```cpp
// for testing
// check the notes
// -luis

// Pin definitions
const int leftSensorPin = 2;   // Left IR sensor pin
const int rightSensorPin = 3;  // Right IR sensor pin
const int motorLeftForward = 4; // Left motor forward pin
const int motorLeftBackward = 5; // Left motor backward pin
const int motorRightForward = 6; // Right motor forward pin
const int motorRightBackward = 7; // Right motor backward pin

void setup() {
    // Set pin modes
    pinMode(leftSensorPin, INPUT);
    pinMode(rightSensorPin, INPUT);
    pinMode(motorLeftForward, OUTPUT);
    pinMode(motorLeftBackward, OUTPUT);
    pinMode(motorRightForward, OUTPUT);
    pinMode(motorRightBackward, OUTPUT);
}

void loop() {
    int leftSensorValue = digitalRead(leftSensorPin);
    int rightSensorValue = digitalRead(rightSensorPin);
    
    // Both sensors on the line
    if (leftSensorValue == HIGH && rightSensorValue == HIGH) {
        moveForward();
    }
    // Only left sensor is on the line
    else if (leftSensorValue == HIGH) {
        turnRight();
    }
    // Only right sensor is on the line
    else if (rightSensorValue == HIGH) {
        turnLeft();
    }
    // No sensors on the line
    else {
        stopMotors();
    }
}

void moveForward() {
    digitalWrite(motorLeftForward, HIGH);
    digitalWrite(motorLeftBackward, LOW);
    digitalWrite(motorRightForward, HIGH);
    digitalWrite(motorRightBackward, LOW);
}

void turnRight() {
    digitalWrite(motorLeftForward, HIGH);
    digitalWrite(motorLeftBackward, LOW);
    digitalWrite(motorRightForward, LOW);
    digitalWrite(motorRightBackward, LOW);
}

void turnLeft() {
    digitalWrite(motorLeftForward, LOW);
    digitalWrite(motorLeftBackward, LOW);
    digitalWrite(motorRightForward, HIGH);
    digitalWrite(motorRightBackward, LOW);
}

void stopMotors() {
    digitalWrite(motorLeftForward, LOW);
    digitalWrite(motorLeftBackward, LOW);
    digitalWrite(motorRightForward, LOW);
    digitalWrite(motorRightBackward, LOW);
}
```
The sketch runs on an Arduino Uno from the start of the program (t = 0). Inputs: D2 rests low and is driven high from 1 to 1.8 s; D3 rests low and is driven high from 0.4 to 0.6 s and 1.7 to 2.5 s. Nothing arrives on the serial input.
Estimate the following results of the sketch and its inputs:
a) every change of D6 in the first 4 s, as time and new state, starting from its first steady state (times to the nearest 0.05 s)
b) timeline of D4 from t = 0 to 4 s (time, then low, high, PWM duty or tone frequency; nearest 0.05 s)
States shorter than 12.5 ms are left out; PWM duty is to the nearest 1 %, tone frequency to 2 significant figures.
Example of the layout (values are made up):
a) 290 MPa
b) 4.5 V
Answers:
a) 0 s low; 0.4 s high; 0.6 s low; 1.7 s high; 2.5 s low
b) 0 s low; 1 s high; 1.8 s low
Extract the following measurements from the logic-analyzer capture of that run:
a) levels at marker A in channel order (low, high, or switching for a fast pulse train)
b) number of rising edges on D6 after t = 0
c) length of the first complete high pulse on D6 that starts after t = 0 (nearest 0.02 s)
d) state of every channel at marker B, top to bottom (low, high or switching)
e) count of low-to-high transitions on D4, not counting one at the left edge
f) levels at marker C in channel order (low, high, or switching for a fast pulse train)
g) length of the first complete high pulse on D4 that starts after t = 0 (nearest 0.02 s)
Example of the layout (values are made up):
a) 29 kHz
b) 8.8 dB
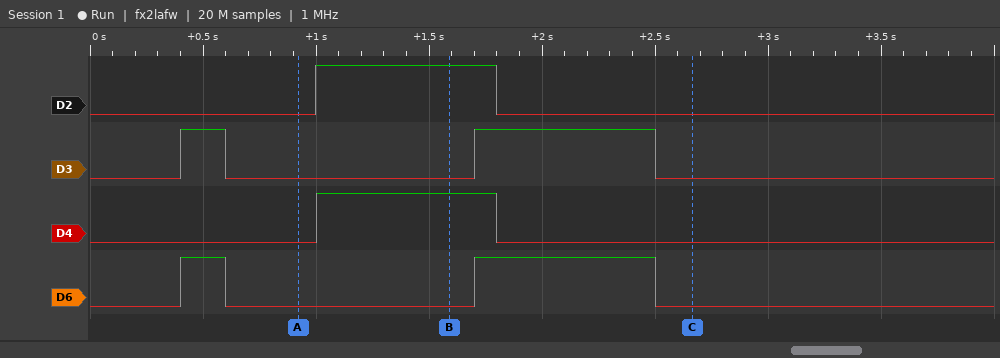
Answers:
a) D2 low, D3 low, D4 low, D6 low
b) 2
c) 0.20 s
d) D2 high, D3 low, D4 high, D6 low
e) 1
f) D2 low, D3 low, D4 low, D6 low
g) 0.80 s
